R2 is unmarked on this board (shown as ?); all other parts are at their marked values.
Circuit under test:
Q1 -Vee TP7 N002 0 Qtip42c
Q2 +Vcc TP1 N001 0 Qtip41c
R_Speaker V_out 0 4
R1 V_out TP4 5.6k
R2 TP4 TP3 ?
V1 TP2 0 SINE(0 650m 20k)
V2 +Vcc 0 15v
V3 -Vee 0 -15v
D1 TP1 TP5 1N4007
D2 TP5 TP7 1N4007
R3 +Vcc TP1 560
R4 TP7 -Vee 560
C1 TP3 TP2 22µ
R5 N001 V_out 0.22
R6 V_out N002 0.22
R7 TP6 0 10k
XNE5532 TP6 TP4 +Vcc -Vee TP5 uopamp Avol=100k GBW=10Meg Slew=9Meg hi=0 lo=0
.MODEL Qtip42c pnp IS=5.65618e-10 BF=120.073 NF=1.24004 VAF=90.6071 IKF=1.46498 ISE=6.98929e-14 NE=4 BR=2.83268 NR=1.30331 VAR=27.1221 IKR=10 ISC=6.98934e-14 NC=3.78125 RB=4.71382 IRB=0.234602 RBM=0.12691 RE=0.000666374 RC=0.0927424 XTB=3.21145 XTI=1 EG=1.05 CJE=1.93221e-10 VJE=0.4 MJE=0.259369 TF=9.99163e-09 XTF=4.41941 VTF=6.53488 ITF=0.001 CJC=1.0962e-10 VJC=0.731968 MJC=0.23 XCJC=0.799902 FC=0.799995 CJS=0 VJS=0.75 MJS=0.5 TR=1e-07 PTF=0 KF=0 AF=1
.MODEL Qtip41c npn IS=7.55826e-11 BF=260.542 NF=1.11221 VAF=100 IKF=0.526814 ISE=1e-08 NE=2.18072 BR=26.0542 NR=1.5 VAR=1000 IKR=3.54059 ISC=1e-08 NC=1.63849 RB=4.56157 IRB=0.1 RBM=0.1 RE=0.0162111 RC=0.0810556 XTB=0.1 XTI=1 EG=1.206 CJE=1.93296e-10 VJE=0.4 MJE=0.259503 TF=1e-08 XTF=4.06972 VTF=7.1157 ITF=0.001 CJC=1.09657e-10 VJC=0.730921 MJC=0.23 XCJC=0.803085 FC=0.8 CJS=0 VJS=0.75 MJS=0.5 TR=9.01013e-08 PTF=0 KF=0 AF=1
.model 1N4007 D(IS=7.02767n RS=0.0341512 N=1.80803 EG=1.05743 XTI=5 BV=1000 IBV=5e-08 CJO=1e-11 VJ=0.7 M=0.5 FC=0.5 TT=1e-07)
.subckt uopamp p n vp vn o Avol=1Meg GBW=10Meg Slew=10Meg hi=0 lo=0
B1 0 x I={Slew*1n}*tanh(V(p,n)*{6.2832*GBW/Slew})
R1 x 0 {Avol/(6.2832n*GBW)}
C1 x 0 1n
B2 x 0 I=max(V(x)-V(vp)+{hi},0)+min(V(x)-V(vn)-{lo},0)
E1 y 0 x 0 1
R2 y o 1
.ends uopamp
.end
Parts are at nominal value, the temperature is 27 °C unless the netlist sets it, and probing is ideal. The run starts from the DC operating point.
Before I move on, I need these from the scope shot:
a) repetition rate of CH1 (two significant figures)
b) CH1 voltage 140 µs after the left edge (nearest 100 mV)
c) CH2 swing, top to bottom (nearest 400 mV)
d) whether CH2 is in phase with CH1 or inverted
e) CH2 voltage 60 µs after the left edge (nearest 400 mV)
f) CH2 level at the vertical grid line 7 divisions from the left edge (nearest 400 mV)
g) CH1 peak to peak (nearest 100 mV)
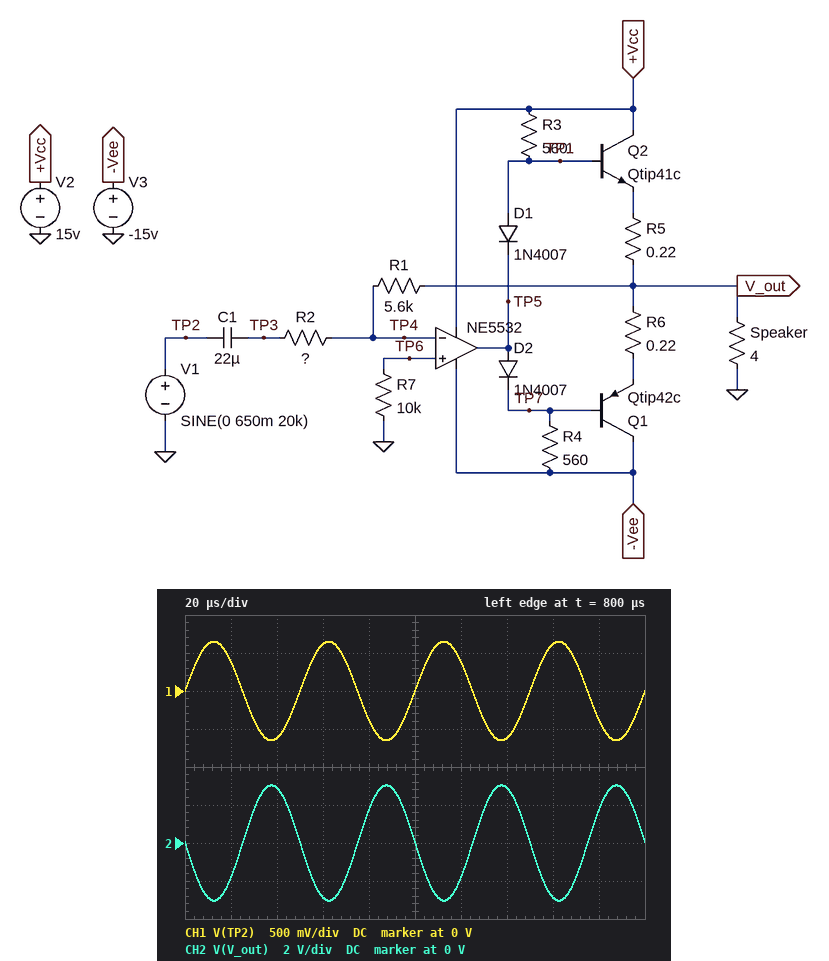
20 kHz
-600 mV
6.0 V
inverted
-2.8 V
2.8 V
1.3 V
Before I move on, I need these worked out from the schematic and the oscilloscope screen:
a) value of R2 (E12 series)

1.2 kΩ
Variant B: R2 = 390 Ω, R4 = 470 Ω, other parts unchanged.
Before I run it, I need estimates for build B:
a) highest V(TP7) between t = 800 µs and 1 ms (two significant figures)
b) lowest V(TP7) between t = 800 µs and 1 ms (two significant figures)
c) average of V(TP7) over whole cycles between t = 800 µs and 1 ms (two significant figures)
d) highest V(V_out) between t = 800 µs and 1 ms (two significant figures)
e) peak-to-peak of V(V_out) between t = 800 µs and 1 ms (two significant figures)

14 V
-6.3 V
2.4 V
4.9 V
10 V
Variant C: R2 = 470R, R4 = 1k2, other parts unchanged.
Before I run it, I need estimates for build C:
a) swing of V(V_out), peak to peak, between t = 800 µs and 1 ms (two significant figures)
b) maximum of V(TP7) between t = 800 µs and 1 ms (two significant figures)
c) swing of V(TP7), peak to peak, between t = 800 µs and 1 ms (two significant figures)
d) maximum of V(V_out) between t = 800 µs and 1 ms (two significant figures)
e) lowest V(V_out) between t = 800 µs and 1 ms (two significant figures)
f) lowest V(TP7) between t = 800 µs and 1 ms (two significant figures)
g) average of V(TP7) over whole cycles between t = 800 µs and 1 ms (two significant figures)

8.1 V
14 V
18 V
4.9 V
-3.2 V
-4.1 V
2.7 V
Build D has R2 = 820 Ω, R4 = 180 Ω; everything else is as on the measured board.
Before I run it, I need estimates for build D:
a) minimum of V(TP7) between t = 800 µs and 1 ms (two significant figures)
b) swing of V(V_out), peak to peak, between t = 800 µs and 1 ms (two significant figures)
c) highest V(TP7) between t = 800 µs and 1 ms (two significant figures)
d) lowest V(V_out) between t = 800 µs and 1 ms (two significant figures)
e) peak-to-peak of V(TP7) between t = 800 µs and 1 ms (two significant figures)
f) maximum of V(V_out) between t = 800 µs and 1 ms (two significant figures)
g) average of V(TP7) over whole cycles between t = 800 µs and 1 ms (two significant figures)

-5.4 V
8.9 V
4.1 V
-4.4 V
9.5 V
4.4 V
-710 mV
